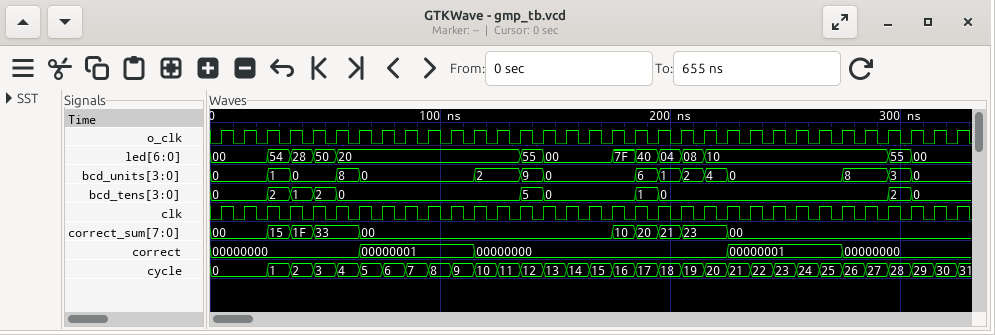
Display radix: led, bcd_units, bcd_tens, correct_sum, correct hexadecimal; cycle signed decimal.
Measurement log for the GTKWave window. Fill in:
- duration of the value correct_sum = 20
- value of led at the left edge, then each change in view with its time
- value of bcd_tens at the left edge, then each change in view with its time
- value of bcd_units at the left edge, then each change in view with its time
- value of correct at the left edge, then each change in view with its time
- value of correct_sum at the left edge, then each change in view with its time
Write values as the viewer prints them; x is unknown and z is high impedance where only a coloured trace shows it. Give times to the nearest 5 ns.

10 ns
00, 54 at 25 ns, 28 at 35 ns, 50 at 45 ns, 20 at 55 ns, 55 at 135 ns, 00 at 145 ns, 7F at 175 ns, 40 at 185 ns, 04 at 195 ns, 08 at 205 ns, 10 at 215 ns, 55 at 295 ns, 00 at 305 ns
0, 2 at 25 ns, 1 at 35 ns, 2 at 45 ns, 0 at 55 ns, 5 at 135 ns, 0 at 145 ns, 1 at 185 ns, 0 at 195 ns, 2 at 295 ns, 0 at 305 ns
0, 1 at 25 ns, 0 at 35 ns, 8 at 55 ns, 0 at 65 ns, 2 at 115 ns, 9 at 135 ns, 0 at 145 ns, 6 at 185 ns, 1 at 195 ns, 2 at 205 ns, 4 at 215 ns, 0 at 225 ns, 8 at 275 ns, 3 at 295 ns, 0 at 305 ns
00000000, 00000001 at 65 ns, 00000000 at 115 ns, 00000001 at 225 ns, 00000000 at 275 ns
00, 15 at 25 ns, 1F at 35 ns, 33 at 45 ns, 00 at 65 ns, 10 at 175 ns, 20 at 185 ns, 21 at 195 ns, 23 at 205 ns, 00 at 225 ns
